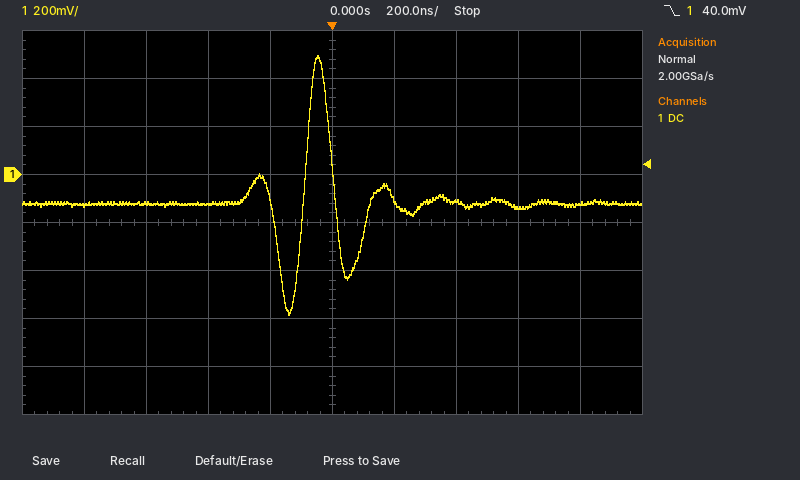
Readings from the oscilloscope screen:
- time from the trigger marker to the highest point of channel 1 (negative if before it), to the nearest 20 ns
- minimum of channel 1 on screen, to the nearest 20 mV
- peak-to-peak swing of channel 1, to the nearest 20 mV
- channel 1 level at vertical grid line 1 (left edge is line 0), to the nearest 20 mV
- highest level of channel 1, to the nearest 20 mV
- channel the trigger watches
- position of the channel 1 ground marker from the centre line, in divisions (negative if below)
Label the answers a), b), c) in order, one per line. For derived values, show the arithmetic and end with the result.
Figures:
a) -40 ns
b) -580 mV
c) 500 mV − (-580 mV) = 1.08 V
d) -120 mV
e) 500 mV
f) channel 1
g) +1.0 div
